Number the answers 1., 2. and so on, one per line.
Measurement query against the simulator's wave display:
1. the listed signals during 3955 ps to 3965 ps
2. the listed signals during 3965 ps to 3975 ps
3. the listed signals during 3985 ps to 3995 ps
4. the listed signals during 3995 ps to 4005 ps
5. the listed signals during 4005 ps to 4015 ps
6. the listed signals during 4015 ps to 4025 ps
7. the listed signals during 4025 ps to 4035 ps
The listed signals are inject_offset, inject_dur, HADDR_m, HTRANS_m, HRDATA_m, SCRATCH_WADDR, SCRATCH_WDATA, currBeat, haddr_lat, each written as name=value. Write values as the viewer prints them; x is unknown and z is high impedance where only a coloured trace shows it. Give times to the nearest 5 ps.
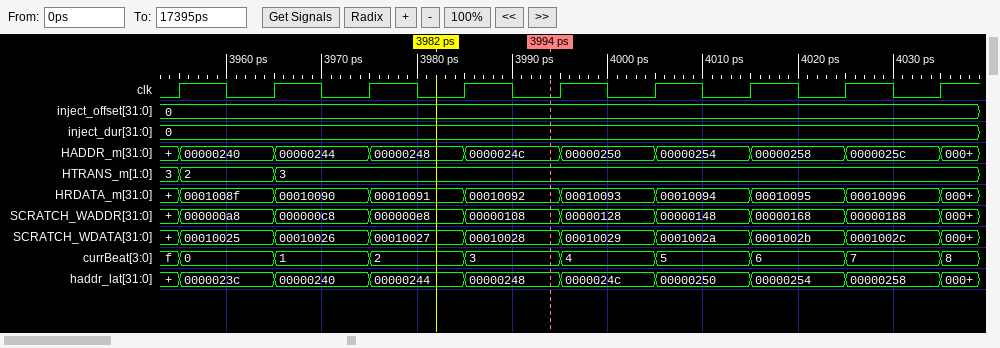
1. inject_offset=0, inject_dur=0, HADDR_m=00000240, HTRANS_m=2, HRDATA_m=0001008f, SCRATCH_WADDR=000000a8, SCRATCH_WDATA=00010025, currBeat=0, haddr_lat=0000023c
2. inject_offset=0, inject_dur=0, HADDR_m=00000244, HTRANS_m=3, HRDATA_m=00010090, SCRATCH_WADDR=000000c8, SCRATCH_WDATA=00010026, currBeat=1, haddr_lat=00000240
3. inject_offset=0, inject_dur=0, HADDR_m=0000024c, HTRANS_m=3, HRDATA_m=00010092, SCRATCH_WADDR=00000108, SCRATCH_WDATA=00010028, currBeat=3, haddr_lat=00000248
4. inject_offset=0, inject_dur=0, HADDR_m=00000250, HTRANS_m=3, HRDATA_m=00010093, SCRATCH_WADDR=00000128, SCRATCH_WDATA=00010029, currBeat=4, haddr_lat=0000024c
5. inject_offset=0, inject_dur=0, HADDR_m=00000254, HTRANS_m=3, HRDATA_m=00010094, SCRATCH_WADDR=00000148, SCRATCH_WDATA=0001002a, currBeat=5, haddr_lat=00000250
6. inject_offset=0, inject_dur=0, HADDR_m=00000258, HTRANS_m=3, HRDATA_m=00010095, SCRATCH_WADDR=00000168, SCRATCH_WDATA=0001002b, currBeat=6, haddr_lat=00000254
7. inject_offset=0, inject_dur=0, HADDR_m=0000025c, HTRANS_m=3, HRDATA_m=00010096, SCRATCH_WADDR=00000188, SCRATCH_WDATA=0001002c, currBeat=7, haddr_lat=00000258
